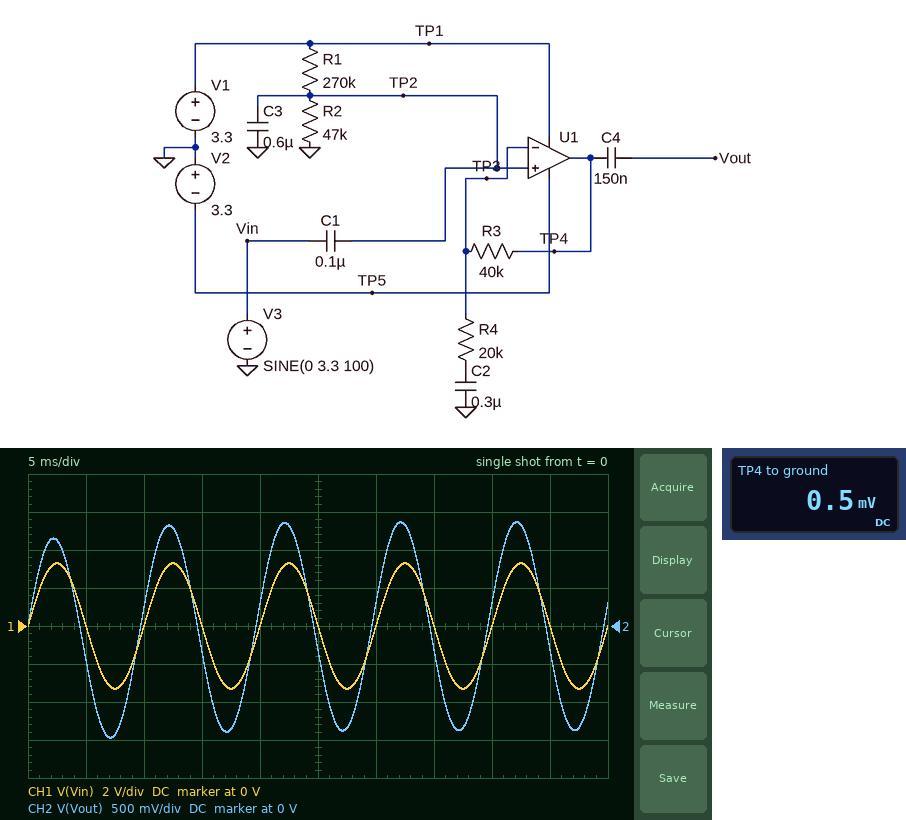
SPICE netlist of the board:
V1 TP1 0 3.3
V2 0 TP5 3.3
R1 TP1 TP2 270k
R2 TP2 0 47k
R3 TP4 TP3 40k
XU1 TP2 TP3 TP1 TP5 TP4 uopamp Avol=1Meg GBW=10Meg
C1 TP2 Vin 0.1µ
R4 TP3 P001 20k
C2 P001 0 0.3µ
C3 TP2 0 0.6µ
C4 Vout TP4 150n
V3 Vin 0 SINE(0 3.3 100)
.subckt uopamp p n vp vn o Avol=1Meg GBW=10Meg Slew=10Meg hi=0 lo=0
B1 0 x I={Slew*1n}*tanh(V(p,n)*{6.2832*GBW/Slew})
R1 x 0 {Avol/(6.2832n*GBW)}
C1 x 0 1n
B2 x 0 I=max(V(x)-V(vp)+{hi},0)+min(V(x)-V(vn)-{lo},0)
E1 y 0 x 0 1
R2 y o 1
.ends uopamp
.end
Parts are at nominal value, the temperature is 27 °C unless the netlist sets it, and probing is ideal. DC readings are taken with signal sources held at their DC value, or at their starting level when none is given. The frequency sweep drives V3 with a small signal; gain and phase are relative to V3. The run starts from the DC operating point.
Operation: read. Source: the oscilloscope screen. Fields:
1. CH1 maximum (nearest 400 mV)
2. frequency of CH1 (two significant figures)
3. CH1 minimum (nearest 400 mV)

3.2 V
100 Hz
-3.2 V
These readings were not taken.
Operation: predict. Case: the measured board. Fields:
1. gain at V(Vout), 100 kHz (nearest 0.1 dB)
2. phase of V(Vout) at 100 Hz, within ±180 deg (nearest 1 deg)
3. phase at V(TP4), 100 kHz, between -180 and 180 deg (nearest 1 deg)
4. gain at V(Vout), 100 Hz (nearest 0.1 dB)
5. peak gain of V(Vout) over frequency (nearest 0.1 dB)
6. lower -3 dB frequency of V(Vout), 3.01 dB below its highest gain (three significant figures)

-7.4 dB
13 deg
-2 deg
-7.6 dB
-7.4 dB
24.8 Hz
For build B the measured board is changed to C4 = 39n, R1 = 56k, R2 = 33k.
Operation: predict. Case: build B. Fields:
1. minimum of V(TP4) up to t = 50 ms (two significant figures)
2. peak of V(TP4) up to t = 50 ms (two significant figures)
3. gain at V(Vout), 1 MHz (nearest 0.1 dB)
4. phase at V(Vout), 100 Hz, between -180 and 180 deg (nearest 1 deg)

-250 mV
2.6 V
-7.7 dB
16 deg
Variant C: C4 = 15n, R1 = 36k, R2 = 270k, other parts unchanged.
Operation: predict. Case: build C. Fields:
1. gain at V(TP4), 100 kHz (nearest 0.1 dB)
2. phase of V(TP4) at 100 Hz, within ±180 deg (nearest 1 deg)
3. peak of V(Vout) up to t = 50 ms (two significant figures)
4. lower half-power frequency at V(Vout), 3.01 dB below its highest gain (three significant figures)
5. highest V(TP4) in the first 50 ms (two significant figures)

-7.4 dB
14 deg
400 mV
25.6 Hz
3.3 V
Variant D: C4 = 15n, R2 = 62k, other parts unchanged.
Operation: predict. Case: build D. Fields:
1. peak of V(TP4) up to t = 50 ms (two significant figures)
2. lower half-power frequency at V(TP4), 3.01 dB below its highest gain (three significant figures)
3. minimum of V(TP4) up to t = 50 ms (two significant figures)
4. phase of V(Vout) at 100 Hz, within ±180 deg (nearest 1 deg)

2.0 V
24.3 Hz
-850 mV
12 deg
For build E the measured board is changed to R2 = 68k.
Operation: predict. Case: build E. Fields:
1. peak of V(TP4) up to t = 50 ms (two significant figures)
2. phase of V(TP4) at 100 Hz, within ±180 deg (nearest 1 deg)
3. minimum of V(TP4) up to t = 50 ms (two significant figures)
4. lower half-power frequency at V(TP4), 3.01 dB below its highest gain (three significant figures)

2.0 V
12 deg
-800 mV
24.2 Hz
